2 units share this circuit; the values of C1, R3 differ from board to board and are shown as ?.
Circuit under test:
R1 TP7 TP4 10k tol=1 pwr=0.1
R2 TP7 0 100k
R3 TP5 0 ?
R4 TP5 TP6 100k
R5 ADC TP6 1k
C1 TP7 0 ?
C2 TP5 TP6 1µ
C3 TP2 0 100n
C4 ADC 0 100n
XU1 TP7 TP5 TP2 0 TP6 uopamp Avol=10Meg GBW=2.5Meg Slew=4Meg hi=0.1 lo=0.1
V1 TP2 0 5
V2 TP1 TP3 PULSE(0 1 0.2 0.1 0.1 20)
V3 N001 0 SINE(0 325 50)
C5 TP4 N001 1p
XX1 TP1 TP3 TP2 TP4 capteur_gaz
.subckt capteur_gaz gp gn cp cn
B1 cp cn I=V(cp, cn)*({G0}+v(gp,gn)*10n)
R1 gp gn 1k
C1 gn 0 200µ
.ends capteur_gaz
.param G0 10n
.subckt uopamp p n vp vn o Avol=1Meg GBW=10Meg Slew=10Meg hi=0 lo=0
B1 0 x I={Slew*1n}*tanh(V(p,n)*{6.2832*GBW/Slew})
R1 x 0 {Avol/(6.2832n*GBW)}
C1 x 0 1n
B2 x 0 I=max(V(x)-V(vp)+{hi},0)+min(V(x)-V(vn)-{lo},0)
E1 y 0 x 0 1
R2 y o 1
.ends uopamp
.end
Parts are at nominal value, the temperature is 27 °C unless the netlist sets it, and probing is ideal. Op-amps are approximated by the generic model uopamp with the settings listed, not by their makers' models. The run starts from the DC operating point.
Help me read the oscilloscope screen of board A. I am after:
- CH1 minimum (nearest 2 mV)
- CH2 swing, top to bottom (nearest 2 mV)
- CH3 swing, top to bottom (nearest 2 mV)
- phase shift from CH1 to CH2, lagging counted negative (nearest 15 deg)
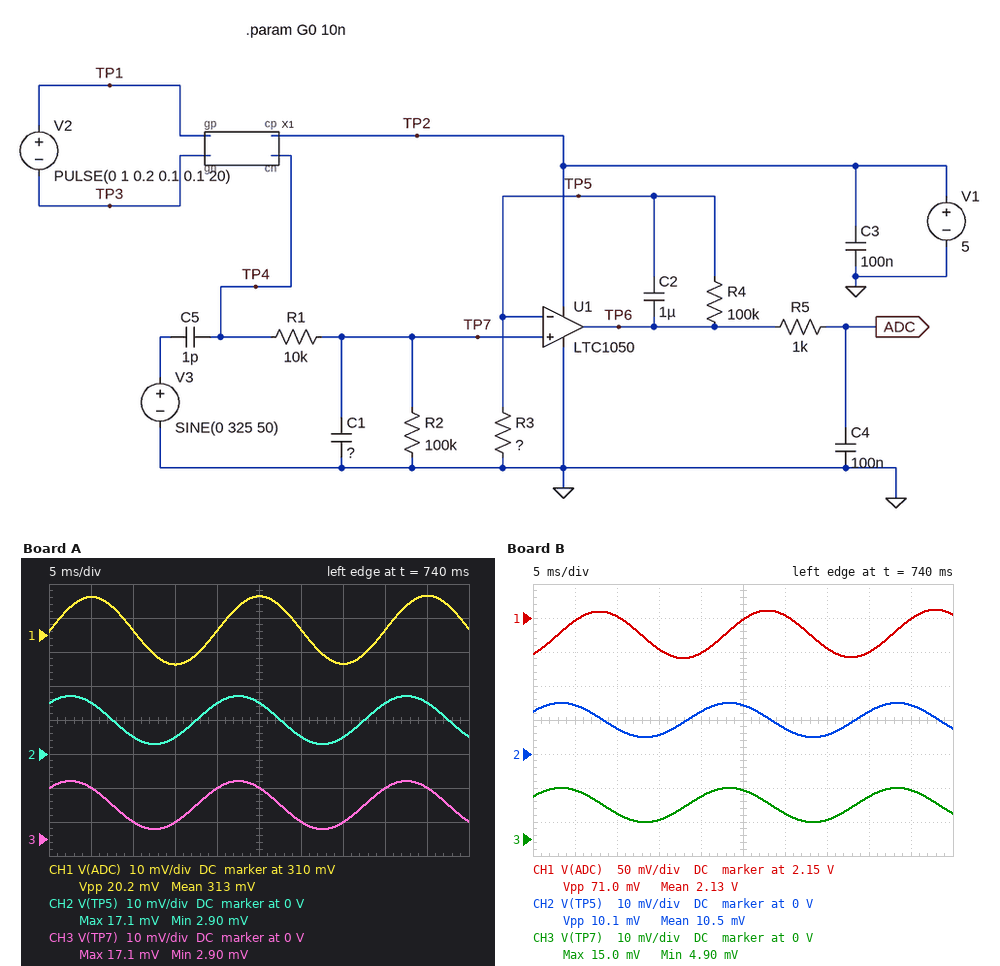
302 mV
14 mV
14 mV
45 deg
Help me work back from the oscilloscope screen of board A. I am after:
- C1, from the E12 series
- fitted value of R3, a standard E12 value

33 nF
3.3 kΩ
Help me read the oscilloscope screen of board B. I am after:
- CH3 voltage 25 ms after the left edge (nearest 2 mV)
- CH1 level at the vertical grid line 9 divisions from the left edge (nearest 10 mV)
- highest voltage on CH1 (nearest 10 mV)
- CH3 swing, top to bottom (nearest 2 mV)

14 mV
2.15 V
2.16 V
10 mV
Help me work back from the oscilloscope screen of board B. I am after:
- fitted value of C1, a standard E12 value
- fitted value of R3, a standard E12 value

56 nF
470 Ω
